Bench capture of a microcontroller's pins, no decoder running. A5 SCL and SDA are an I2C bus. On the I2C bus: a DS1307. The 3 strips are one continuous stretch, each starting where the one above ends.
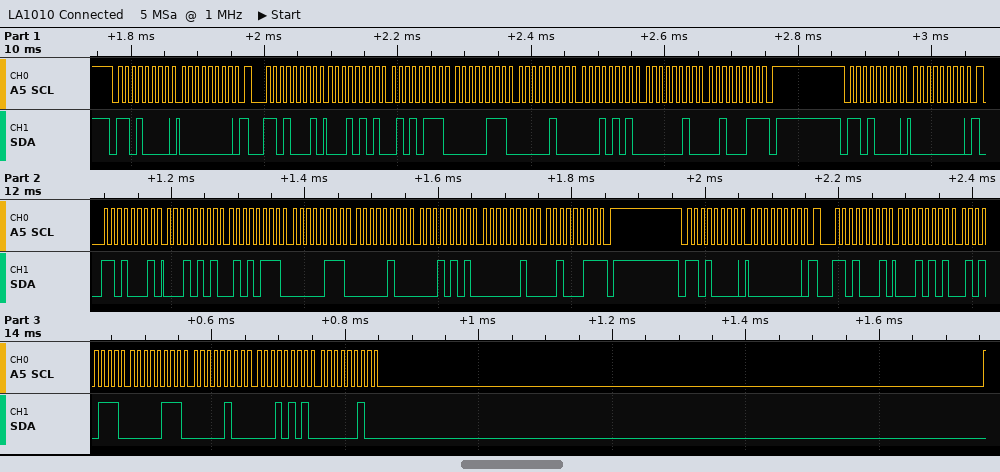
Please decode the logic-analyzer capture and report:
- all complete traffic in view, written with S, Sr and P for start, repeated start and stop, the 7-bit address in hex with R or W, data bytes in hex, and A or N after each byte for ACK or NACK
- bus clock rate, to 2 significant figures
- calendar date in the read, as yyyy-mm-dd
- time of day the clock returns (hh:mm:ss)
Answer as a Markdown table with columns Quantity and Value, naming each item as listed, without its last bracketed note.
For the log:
| Quantity | Value |
|---|---|
| all complete traffic in view, written with S, Sr and P for start, repeated start and stop, the 7-bit address in hex with R or W, data bytes in hex, and A or N after each byte for ACK or NACK | S 68W A 00 A Sr 68R A 15 A 57 A 07 A 04 A 15 A 02 A 23 N P S 68W A 00 A Sr 68R A 15 A 57 A 07 A 04 A 15 A 02 A 23 N P S 68W A 00 A Sr 68R A 15 A 57 A 07 A 04 A 15 A 02 A |
| bus clock rate, to 2 significant figures | 100 kHz |
| calendar date in the read, as yyyy-mm-dd | 2023-02-15 |
| time of day the clock returns | 07:57:15 |
